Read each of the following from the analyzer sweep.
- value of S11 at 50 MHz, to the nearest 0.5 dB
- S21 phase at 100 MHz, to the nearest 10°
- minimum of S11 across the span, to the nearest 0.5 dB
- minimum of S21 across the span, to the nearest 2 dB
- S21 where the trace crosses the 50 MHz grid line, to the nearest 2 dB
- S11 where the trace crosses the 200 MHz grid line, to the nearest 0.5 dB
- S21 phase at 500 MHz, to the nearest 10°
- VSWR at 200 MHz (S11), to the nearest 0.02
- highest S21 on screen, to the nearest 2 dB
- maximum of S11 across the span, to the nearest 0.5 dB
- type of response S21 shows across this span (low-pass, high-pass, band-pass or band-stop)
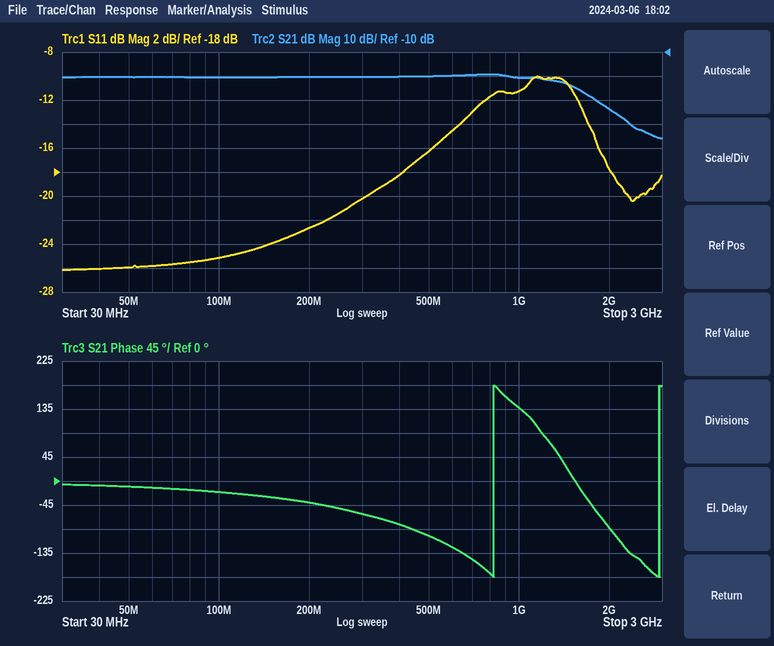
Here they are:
-26.0 dB
-20°
-26.0 dB
-46 dB
-20 dB
-22.5 dB
-100°
1.16
-20 dB
-10.0 dB
low-pass
